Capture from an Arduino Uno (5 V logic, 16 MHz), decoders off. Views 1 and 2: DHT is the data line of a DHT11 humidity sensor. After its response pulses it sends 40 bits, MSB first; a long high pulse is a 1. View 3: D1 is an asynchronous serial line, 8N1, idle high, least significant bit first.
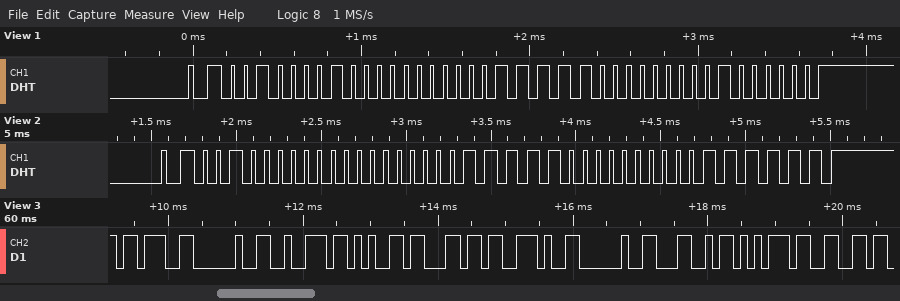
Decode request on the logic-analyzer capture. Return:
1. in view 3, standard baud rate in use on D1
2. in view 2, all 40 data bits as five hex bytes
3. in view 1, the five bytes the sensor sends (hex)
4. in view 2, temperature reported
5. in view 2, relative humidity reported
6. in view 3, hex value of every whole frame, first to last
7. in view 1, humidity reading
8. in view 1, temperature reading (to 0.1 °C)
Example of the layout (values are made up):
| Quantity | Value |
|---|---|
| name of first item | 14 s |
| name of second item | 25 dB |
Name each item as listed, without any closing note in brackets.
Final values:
| Quantity | Value |
|---|---|
| in view 3, standard baud rate in use on D1 | 9600 baud |
| in view 2, all 40 data bits as five hex bytes | 20 00 1F 00 3F |
| in view 1, the five bytes the sensor sends | 21 00 1F 00 40 |
| in view 2, temperature reported | 31.0 °C |
| in view 2, relative humidity reported | 32 % |
| in view 3, hex value of every whole frame, first to last | 0x3B 0x20 0x72 0x65 0x6C 0x2E 0x20 0x4C 0x75 0x66 |
| in view 1, humidity reading | 33 % |
| in view 1, temperature reading | 31.0 °C |
